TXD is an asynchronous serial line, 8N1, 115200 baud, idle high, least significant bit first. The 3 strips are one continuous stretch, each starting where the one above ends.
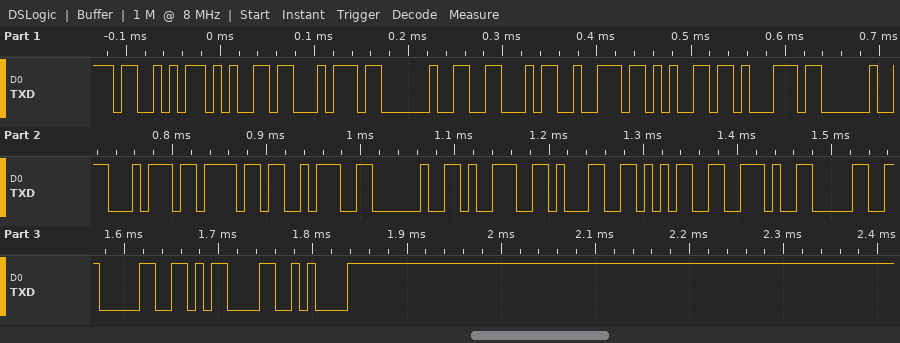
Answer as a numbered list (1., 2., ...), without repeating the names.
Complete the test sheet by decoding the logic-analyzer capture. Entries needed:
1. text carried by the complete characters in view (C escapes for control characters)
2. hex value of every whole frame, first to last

1. "Set Freq to: 915.00\r\n"
2. 53 65 74 20 46 72 65 71 20 74 6F 3A 20 39 31 35 2E 30 30 0D 0A
